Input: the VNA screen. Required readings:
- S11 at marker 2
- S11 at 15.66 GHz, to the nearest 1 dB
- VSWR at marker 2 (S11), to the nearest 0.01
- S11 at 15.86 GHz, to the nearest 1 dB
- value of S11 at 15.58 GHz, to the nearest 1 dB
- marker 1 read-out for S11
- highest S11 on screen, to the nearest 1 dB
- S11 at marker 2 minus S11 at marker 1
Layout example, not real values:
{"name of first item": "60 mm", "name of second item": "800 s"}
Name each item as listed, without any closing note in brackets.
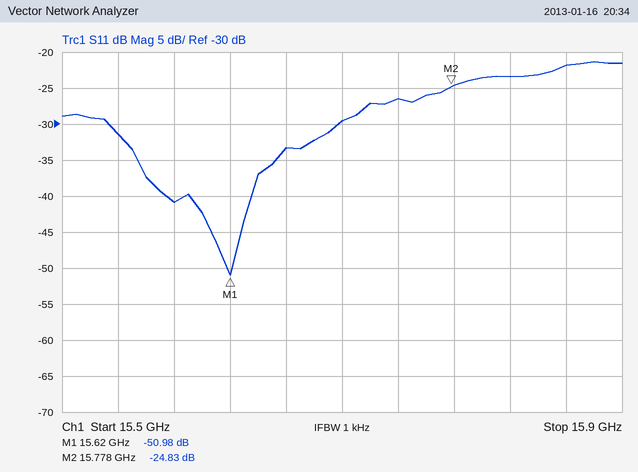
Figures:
{"S11 at marker 2": "-24.83 dB", "S11 at 15.66 GHz, to the nearest 1 dB": "-33 dB", "VSWR at marker 2 (S11), to the nearest 0.01": "1.12", "S11 at 15.86 GHz, to the nearest 1 dB": "-22 dB", "value of S11 at 15.58 GHz, to the nearest 1 dB": "-41 dB", "marker 1 read-out for S11": "-50.98 dB", "highest S11 on screen, to the nearest 1 dB": "-21 dB", "S11 at marker 2 minus S11 at marker 1": "26.15 dB"}
